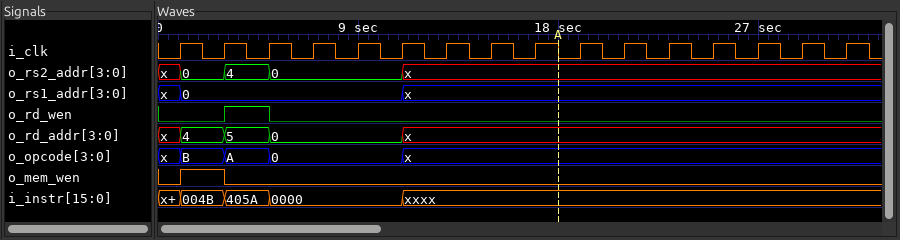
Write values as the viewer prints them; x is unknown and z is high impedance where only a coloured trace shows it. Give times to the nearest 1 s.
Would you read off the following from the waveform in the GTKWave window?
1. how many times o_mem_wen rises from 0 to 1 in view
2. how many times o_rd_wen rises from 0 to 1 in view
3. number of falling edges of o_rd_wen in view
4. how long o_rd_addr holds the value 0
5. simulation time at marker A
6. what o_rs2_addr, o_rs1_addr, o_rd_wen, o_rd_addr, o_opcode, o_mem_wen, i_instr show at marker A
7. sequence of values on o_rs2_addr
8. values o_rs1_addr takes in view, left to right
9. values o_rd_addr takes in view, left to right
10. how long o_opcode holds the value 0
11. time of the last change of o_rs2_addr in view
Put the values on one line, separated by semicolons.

1; 1; 1; 6 s; 18 s; o_rs2_addr=x, o_rs1_addr=x, o_rd_wen=0, o_rd_addr=x, o_opcode=x, o_mem_wen=0, i_instr=xxxx; x, 0, 4, 0, x; x, 0, x; x, 4, 5, 0, x; 6 s; 11 s
